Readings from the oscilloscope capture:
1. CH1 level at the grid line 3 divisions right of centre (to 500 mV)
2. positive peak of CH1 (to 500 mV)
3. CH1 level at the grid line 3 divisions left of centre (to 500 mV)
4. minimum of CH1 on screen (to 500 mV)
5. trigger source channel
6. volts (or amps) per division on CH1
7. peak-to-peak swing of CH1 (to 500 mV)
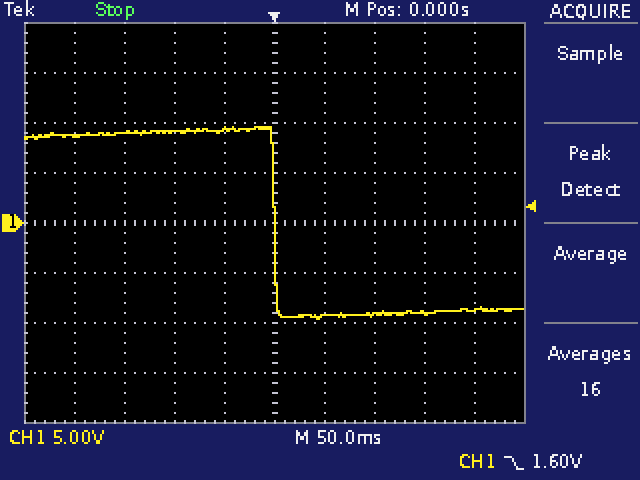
-9.0 V
9.5 V
9.0 V
-9.5 V
CH1
5 V
19.0 V
